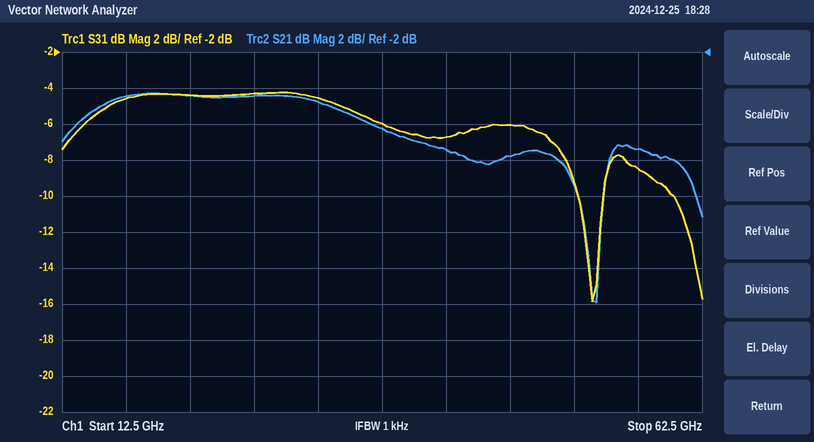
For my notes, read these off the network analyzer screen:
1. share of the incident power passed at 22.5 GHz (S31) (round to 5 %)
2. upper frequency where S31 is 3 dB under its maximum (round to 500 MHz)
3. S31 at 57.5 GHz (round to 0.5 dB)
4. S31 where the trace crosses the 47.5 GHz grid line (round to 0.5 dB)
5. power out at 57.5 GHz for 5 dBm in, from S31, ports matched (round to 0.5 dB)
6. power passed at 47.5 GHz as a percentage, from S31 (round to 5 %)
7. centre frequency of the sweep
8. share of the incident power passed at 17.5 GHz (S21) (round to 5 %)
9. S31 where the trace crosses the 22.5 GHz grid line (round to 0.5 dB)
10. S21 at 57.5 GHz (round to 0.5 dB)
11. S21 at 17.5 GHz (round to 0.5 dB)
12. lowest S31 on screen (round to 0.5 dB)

35 %
51.0 GHz
-8.5 dB
-6.0 dB
-3.5 dBm
25 %
37.5 GHz
35 %
-4.5 dB
-7.5 dB
-4.5 dB
-16.0 dB
